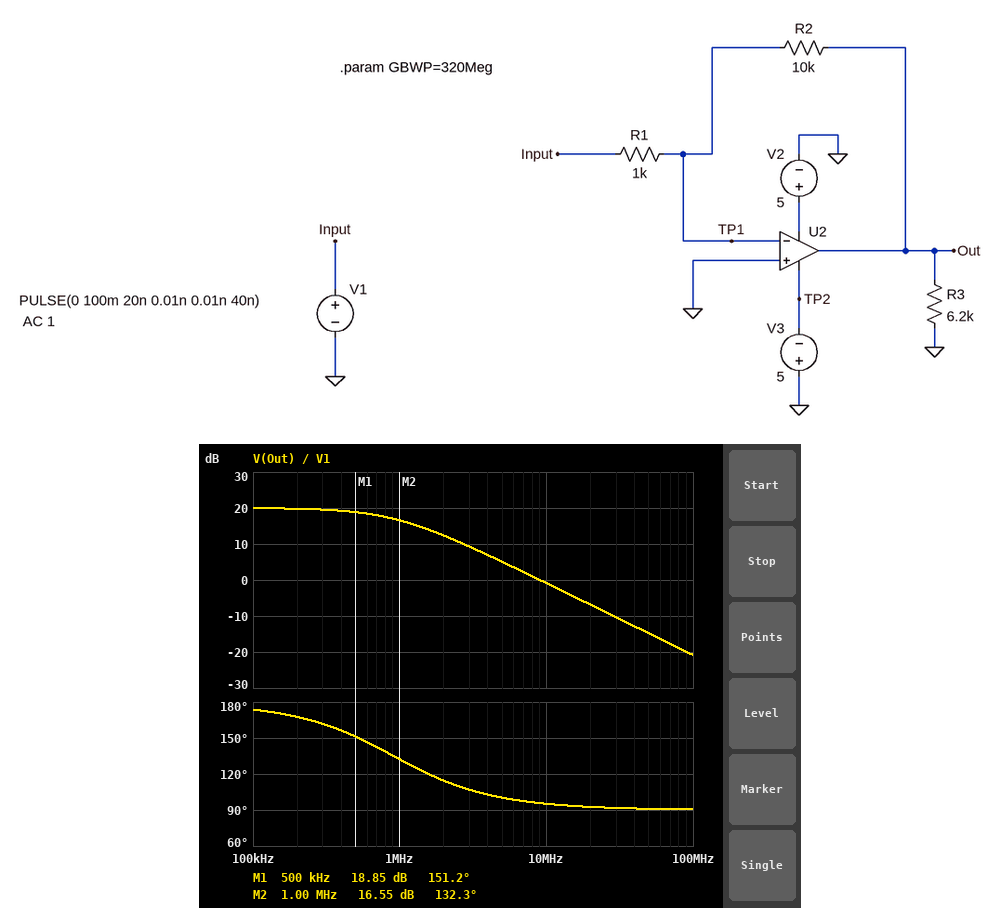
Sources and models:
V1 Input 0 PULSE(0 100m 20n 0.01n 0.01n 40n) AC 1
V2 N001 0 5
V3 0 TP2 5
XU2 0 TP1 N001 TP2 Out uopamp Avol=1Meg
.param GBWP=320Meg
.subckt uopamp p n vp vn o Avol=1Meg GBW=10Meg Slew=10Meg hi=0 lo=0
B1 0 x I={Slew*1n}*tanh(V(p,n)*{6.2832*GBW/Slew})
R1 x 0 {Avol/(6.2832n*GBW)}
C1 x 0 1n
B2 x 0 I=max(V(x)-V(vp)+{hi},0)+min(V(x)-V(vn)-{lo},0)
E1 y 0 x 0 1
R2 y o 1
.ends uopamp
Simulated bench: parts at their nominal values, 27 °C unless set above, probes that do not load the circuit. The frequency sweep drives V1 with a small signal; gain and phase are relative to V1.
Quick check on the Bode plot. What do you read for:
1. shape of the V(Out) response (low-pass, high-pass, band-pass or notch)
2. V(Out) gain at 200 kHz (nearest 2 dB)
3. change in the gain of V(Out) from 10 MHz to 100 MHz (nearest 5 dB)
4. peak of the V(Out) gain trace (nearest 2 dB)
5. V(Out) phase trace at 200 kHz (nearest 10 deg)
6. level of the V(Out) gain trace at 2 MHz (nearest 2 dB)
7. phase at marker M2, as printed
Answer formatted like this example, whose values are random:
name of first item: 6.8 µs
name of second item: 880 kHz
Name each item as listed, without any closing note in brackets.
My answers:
shape of the V(Out) response: low-pass
V(Out) gain at 200 kHz: 20 dB
change in the gain of V(Out) from 10 MHz to 100 MHz: -20 dB
peak of the V(Out) gain trace: 20 dB
V(Out) phase trace at 200 kHz: 170 deg
level of the V(Out) gain trace at 2 MHz: 12 dB
phase at marker M2, as printed: 132.3 deg
